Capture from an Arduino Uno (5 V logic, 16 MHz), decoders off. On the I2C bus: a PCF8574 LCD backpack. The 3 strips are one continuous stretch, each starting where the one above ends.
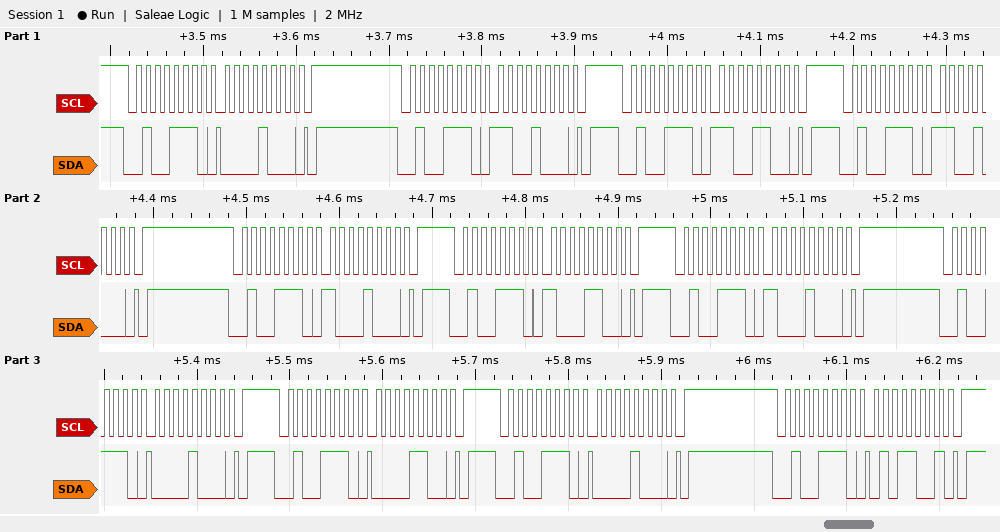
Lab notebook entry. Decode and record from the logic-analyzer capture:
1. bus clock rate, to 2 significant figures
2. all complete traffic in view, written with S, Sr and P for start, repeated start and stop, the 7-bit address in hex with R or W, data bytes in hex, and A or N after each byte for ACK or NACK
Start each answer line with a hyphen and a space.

- 100 kHz
- S 27W A 08 A P S 27W A C8 A P S 27W A CC A P S 27W A C8 A P S 27W A 88 A P S 27W A 8C A P S 27W A 88 A P S 27W A 08 A P S 27W A 0C A P S 27W A 08 A P S 27W A 59 A P
